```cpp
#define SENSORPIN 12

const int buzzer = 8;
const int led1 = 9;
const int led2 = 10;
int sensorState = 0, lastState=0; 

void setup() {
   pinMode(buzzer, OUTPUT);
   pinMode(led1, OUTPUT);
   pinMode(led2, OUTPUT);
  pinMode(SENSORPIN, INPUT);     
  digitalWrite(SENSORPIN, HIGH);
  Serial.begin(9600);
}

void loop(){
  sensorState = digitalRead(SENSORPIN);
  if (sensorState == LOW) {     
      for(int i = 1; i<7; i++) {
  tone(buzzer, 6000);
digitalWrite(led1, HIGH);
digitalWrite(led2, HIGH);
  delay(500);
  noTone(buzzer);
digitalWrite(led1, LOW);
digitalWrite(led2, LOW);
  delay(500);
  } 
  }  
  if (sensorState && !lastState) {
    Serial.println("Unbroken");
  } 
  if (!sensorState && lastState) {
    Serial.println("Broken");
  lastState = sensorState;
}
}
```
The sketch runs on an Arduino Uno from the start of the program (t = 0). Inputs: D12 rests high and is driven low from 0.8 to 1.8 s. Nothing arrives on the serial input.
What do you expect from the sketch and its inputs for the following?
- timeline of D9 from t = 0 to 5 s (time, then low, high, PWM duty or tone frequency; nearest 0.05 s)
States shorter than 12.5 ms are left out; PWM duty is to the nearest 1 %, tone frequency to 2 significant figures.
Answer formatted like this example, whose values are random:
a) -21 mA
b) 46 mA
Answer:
a) 0 s low; 0.8 s high; 1.3 s low; 1.8 s high; 2.3 s low; 2.8 s high; 3.3 s low; 3.8 s high; 4.3 s low; 4.8 s high
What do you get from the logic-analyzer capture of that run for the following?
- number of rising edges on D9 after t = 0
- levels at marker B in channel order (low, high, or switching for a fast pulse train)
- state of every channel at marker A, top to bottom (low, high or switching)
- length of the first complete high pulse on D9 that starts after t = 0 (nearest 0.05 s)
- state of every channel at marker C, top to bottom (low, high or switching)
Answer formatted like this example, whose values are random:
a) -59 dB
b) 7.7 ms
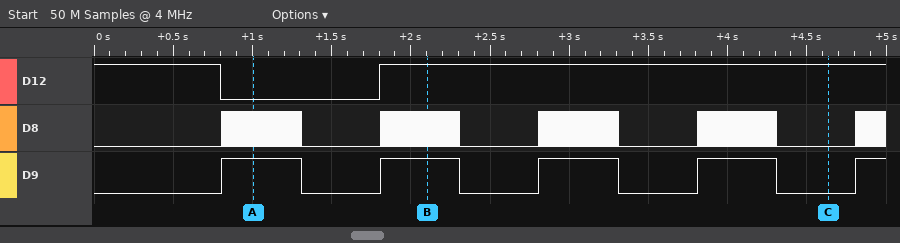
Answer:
a) 5
b) D12 high, D8 switching, D9 high
c) D12 low, D8 switching, D9 high
d) 0.50 s
e) D12 high, D8 low, D9 low
